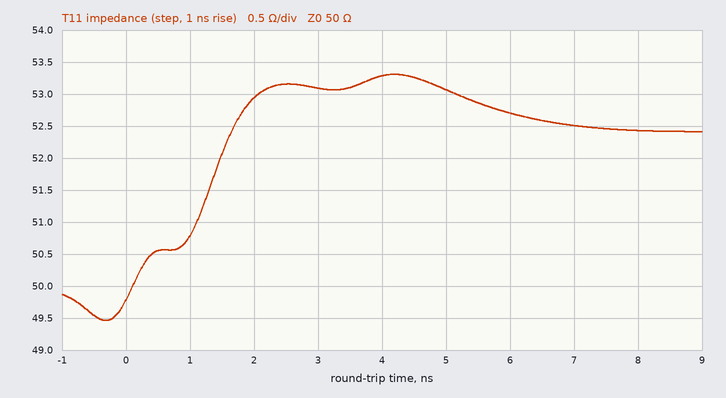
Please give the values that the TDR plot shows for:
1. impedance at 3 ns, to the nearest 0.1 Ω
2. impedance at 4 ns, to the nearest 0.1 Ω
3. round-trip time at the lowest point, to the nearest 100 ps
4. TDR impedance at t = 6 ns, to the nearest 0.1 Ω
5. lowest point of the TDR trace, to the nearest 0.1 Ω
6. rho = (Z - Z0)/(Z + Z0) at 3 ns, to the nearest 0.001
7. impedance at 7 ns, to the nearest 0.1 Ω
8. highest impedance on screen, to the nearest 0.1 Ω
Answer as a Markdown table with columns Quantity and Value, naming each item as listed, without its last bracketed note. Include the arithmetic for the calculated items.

| Quantity | Value |
|---|---|
| impedance at 3 ns, to the nearest 0.1 Ω | 53.1 Ω |
| impedance at 4 ns, to the nearest 0.1 Ω | 53.3 Ω |
| round-trip time at the lowest point, to the nearest 100 ps | -300 ps |
| TDR impedance at t = 6 ns, to the nearest 0.1 Ω | 52.7 Ω |
| lowest point of the TDR trace, to the nearest 0.1 Ω | 49.5 Ω |
| rho = (Z - Z0)/(Z + Z0) at 3 ns, to the nearest 0.001 | (53.1 − 50)/(53.1 + 50) ≈ +0.030 |
| impedance at 7 ns, to the nearest 0.1 Ω | 52.5 Ω |
| highest impedance on screen, to the nearest 0.1 Ω | 53.3 Ω |
